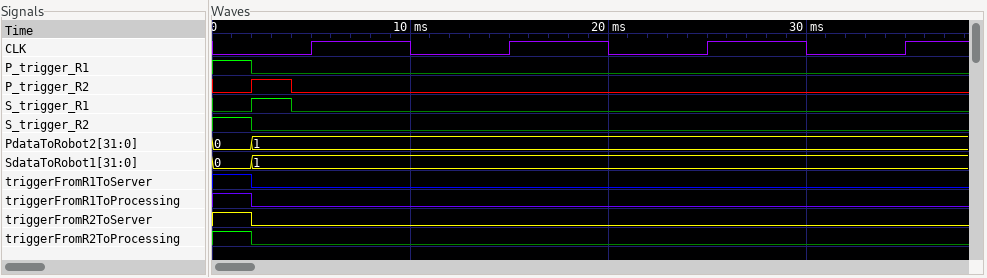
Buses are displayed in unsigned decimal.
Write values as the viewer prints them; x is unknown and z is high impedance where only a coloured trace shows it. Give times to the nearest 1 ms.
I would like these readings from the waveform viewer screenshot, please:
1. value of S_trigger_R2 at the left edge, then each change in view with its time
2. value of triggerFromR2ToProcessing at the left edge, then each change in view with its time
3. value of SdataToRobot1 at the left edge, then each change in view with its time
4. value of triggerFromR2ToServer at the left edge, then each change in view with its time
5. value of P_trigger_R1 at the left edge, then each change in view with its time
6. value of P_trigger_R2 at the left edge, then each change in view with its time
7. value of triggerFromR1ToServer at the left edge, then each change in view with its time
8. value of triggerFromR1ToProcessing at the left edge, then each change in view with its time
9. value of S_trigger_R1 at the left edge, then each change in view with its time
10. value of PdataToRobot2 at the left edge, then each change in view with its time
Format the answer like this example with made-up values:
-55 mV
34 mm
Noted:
1, 0 at 2 ms
1, 0 at 2 ms
0, 1 at 2 ms
1, 0 at 2 ms
1, 0 at 2 ms
0, 1 at 2 ms, 0 at 4 ms
1, 0 at 2 ms
1, 0 at 2 ms
0, 1 at 2 ms, 0 at 4 ms
0, 1 at 2 ms
